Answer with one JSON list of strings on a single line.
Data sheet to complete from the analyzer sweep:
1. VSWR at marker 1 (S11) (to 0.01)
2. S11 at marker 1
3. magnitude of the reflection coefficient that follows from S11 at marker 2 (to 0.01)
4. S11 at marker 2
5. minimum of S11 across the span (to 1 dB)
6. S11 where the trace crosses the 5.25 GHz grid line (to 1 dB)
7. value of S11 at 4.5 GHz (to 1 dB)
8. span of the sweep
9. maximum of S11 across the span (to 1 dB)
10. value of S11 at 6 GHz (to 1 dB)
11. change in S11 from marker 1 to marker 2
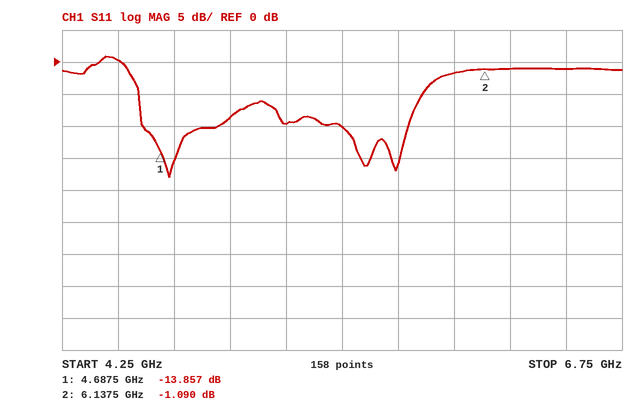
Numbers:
["1.51", "-13.857 dB", "0.88", "-1.090 dB", "-18 dB", "-10 dB", "0 dB", "2.5 GHz", "1 dB", "-2 dB", "12.767 dB"]
